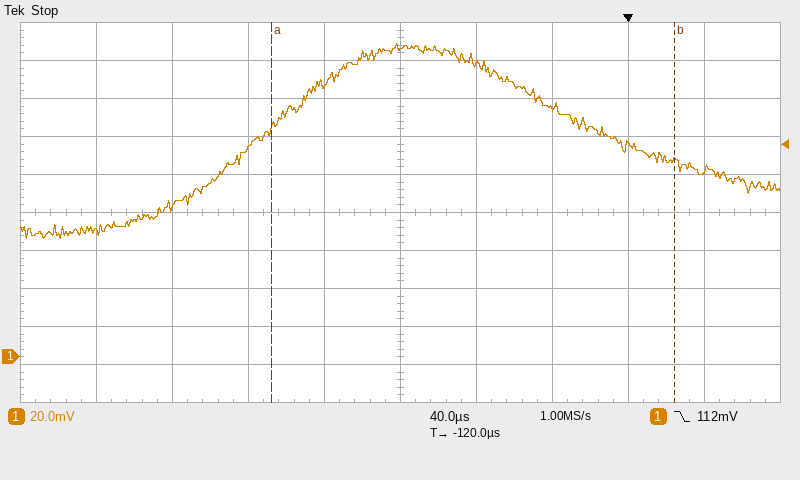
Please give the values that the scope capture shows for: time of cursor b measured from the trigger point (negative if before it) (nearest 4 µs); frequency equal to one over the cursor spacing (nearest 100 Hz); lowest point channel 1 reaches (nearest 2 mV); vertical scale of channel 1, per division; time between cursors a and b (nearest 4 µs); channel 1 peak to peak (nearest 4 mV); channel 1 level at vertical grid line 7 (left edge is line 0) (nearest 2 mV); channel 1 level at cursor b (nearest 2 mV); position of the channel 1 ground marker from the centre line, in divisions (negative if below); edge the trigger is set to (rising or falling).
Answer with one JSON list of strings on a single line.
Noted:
["+24 µs", "4.7 kHz", "62 mV", "20 mV", "212 µs", "104 mV", "132 mV", "104 mV", "-3.8 div", "falling"]
